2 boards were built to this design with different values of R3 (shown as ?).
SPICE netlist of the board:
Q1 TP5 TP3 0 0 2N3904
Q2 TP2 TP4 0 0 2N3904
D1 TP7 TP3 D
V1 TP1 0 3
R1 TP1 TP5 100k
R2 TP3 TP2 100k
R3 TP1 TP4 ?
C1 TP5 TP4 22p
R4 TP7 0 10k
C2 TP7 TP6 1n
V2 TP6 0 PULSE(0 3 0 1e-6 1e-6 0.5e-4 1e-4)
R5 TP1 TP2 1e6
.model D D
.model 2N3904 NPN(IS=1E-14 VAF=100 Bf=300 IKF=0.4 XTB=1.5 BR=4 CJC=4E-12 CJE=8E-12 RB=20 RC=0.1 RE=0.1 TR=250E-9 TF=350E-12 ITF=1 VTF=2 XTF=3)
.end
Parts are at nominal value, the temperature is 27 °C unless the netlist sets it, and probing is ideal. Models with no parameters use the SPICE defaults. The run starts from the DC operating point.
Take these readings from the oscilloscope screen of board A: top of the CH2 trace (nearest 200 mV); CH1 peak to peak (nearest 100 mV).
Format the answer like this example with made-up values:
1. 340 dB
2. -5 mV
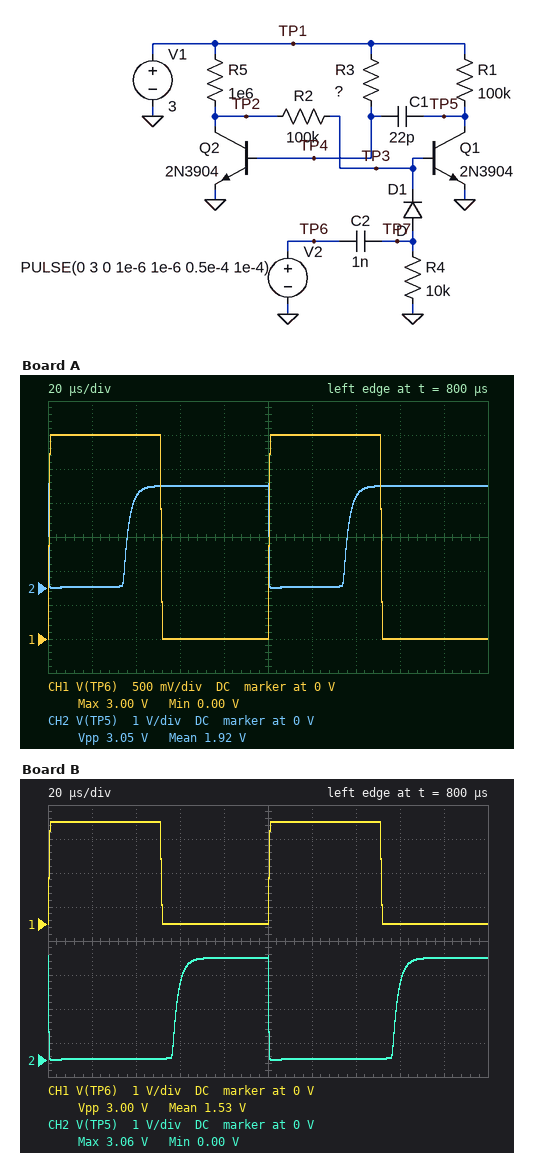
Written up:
1. 3.0 V
2. 3.0 V
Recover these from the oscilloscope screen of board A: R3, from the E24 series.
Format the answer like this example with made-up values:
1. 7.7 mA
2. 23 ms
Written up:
1. 1.8 MΩ
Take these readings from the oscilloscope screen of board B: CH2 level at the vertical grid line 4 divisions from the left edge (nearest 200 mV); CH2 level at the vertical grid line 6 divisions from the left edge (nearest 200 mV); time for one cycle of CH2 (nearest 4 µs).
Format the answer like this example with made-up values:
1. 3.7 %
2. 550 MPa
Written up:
1. 3.0 V
2. 0 V
3. 100 µs
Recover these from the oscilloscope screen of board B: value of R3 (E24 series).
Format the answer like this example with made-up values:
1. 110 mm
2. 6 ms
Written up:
1. 3 MΩ
